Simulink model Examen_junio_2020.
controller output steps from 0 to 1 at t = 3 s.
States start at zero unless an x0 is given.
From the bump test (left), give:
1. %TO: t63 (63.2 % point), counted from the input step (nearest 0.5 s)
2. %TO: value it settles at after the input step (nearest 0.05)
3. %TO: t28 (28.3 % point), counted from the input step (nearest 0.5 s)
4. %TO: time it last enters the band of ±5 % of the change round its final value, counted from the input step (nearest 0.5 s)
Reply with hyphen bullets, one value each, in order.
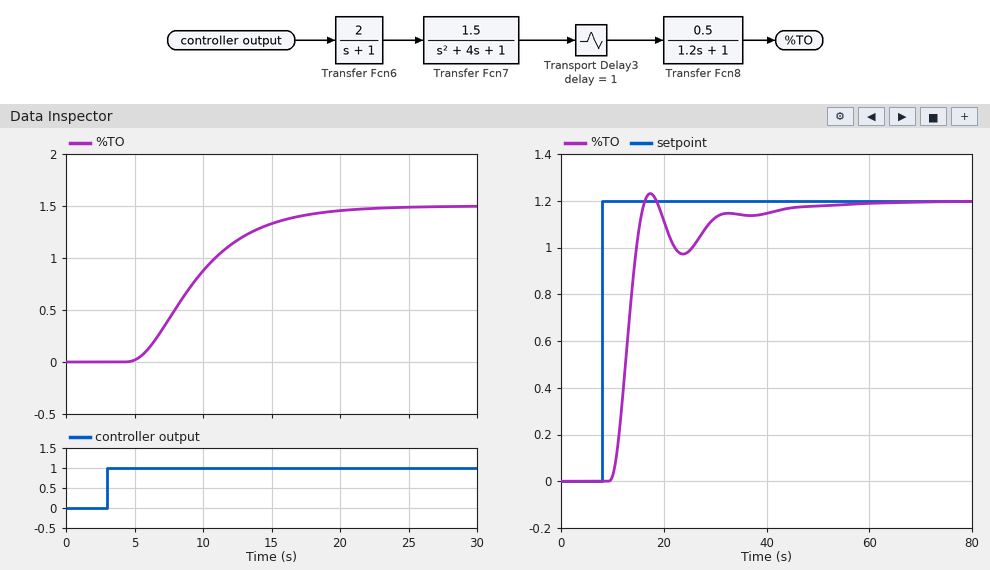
- 7.5 s
- 1.50
- 4.5 s
- 15.0 s
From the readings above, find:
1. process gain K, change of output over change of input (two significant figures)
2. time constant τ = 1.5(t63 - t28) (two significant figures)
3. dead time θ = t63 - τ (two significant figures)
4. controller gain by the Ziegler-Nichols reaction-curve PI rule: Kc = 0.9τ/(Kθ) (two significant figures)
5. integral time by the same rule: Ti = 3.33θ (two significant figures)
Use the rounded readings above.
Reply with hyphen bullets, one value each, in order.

- 1.5
- 4.5 s
- 3.0 s
- 0.90
- 10.0 s
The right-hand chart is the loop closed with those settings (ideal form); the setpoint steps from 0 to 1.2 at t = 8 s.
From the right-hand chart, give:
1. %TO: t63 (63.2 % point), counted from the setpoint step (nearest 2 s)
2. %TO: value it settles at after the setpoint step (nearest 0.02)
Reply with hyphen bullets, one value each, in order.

- 6 s
- 1.20
